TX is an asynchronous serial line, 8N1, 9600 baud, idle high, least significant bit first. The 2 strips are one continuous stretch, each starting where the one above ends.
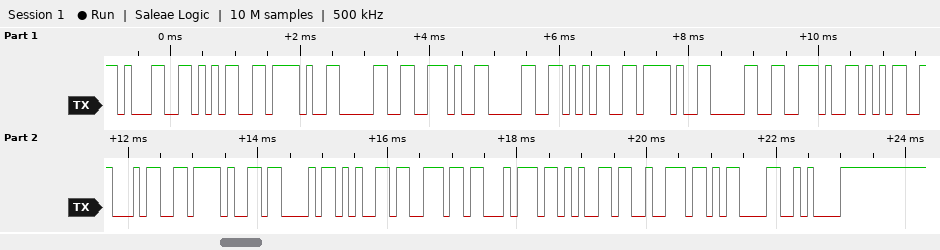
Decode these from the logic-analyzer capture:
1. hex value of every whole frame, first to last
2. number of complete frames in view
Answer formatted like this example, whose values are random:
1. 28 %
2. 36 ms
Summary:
1. 0x31 0x35 0x2F 0x30 0x2E 0x30 0x35 0x2F 0x30 0x2E 0x35 0x34 0x2F 0x43 0x65 0x6E 0x74 0x65 0x72 0x0D 0x0A
2. 21
